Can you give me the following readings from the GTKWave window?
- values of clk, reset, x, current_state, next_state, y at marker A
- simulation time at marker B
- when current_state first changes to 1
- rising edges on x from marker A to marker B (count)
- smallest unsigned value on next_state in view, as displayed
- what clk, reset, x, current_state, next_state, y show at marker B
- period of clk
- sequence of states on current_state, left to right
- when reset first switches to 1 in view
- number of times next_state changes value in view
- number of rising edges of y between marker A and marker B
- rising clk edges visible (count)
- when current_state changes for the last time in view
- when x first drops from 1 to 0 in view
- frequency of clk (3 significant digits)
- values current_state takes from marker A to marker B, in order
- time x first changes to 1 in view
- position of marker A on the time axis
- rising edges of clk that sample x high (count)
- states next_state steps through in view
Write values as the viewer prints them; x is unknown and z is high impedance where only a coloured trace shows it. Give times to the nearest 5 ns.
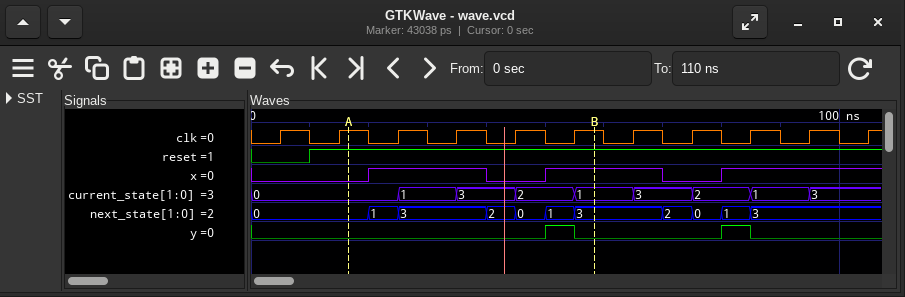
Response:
clk=1, reset=1, x=0, current_state=0, next_state=0, y=0
60 ns
25 ns
2
0
clk=1, reset=1, x=1, current_state=1, next_state=3, y=0
10 ns
0, 1, 3, 2, 1, 3, 2, 1, 3
10 ns
10
1
11
95 ns
40 ns
100 MHz
0, 1, 3, 2, 1
20 ns
15 ns
7
0, 1, 3, 2, 0, 1, 3, 2, 0, 1, 3
